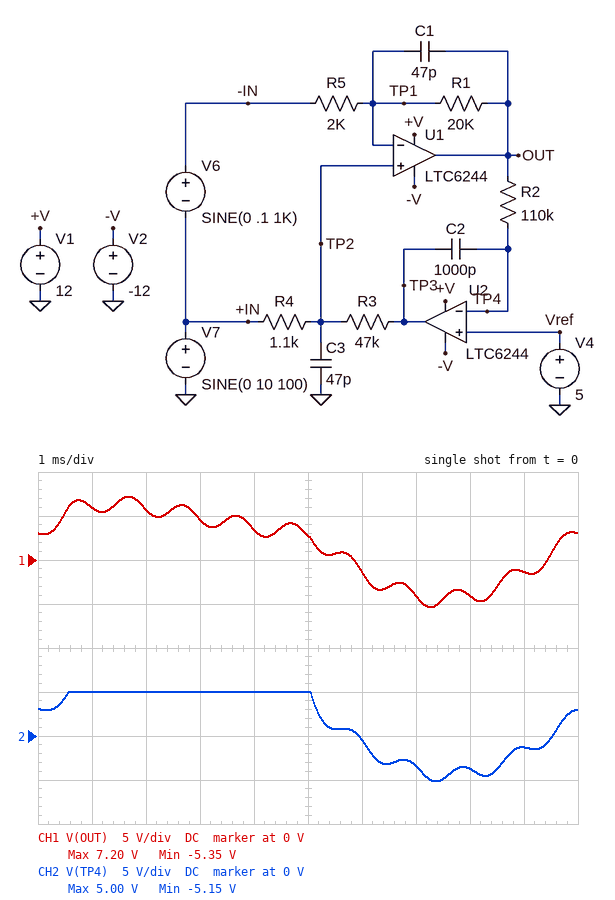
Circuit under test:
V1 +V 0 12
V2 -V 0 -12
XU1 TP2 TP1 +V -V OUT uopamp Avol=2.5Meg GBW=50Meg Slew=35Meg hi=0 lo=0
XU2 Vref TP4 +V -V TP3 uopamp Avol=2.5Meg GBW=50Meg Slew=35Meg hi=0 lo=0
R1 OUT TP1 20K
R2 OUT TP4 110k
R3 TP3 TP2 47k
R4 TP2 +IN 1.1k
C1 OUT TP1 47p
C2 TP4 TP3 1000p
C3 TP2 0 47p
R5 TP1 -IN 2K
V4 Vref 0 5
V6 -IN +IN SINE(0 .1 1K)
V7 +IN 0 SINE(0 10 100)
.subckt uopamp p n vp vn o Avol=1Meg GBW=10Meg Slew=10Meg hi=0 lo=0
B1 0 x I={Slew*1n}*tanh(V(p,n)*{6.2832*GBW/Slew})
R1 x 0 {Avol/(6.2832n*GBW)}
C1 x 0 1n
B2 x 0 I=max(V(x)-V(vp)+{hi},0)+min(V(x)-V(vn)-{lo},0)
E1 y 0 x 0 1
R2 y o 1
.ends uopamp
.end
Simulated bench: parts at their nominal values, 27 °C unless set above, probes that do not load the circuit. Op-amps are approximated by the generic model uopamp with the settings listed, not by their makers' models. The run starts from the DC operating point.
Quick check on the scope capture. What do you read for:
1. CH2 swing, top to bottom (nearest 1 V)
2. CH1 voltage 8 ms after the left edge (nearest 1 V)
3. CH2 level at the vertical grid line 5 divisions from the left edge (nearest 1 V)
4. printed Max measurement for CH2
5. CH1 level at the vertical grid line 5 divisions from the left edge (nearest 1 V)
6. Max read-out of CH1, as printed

10 V
-4 V
5 V
5.00 V
3 V
7.20 V
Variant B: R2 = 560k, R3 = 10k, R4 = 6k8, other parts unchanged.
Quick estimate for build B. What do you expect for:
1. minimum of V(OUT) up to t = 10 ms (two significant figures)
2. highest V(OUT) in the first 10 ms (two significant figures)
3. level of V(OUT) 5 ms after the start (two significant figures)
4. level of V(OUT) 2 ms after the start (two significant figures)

1.8 V
8.2 V
7.2 V
3.5 V
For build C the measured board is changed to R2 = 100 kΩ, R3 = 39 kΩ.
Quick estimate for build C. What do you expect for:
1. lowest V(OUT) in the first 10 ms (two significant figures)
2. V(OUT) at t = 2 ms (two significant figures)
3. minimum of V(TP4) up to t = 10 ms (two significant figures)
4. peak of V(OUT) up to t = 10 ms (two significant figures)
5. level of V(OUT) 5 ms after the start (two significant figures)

-4.3 V
5.3 V
-4.1 V
6.8 V
3.2 V
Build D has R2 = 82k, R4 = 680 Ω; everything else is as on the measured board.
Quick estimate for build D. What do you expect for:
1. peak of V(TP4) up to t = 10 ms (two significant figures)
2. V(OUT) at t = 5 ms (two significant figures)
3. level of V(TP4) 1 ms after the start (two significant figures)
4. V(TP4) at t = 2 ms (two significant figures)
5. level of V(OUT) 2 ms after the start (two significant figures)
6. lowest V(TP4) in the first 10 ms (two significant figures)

7.3 V
1.9 V
5.0 V
5.3 V
6.1 V
-7.3 V
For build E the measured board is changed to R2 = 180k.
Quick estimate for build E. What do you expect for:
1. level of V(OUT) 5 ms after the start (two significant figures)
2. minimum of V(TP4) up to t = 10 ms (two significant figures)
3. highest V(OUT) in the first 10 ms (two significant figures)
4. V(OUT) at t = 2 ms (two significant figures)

2.0 V
-5.0 V
7.9 V
6.5 V
